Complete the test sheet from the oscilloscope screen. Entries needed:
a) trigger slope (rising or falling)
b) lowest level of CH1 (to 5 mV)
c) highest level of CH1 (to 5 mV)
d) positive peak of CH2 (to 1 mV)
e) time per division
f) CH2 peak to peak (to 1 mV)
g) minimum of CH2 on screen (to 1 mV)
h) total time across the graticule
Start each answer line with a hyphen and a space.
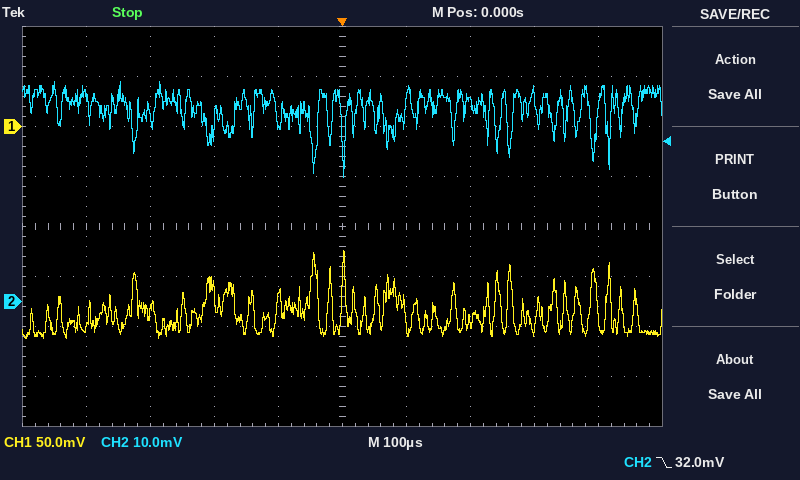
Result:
- falling
- -210 mV
- -125 mV
- 44 mV
- 100 µs
- 19 mV
- 25 mV
- 1 ms
